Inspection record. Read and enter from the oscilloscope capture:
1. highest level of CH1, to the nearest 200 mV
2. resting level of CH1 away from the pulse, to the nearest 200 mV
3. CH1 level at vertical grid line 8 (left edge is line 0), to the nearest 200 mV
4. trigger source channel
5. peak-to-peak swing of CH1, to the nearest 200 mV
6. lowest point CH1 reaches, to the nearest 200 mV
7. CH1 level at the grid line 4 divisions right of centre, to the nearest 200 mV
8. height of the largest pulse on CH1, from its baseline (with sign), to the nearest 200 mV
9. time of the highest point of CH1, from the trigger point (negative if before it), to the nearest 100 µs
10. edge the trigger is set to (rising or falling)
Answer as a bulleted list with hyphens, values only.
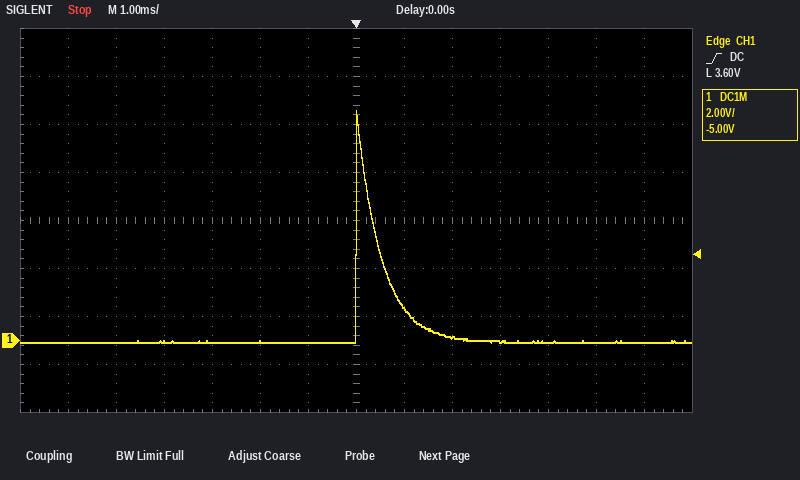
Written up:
- 9.6 V
- 0.0 V
- 1.4 V
- CH1
- 9.6 V
- 0.0 V
- 0.0 V
- +9.6 V
- 0.0 ms
- rising
